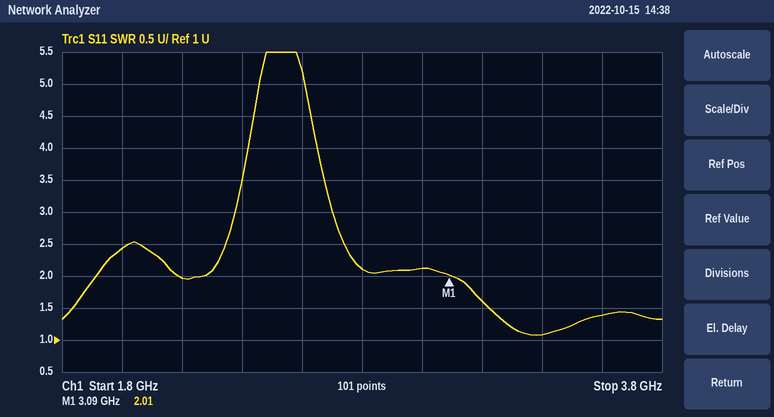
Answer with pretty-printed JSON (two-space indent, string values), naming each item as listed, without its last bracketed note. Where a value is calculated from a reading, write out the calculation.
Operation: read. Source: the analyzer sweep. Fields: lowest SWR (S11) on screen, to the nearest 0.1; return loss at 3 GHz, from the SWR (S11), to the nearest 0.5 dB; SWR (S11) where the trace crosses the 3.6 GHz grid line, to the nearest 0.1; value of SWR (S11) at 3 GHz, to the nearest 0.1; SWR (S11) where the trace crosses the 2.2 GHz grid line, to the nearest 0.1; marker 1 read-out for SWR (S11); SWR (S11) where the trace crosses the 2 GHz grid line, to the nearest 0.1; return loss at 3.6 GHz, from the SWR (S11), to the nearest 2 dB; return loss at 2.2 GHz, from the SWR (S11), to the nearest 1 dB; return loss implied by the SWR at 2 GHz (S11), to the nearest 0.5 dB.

{
  "lowest SWR (S11) on screen, to the nearest 0.1": "1.1",
  "return loss at 3 GHz, from the SWR (S11), to the nearest 0.5 dB": "−20 log10((2.1 − 1)/(2.1 + 1)) ≈ 9.0 dB",
  "SWR (S11) where the trace crosses the 3.6 GHz grid line, to the nearest 0.1": "1.4",
  "value of SWR (S11) at 3 GHz, to the nearest 0.1": "2.1",
  "SWR (S11) where the trace crosses the 2.2 GHz grid line, to the nearest 0.1": "2.0",
  "marker 1 read-out for SWR": "2.01",
  "SWR (S11) where the trace crosses the 2 GHz grid line, to the nearest 0.1": "2.4",
  "return loss at 3.6 GHz, from the SWR (S11), to the nearest 2 dB": "−20 log10((1.4 − 1)/(1.4 + 1)) ≈ 16 dB",
  "return loss at 2.2 GHz, from the SWR (S11), to the nearest 1 dB": "−20 log10((2 − 1)/(2 + 1)) ≈ 10 dB",
  "return loss implied by the SWR at 2 GHz (S11), to the nearest 0.5 dB": "−20 log10((2.4 − 1)/(2.4 + 1)) ≈ 7.71 dB, so 7.5 dB to the nearest 0.5 dB"
}
